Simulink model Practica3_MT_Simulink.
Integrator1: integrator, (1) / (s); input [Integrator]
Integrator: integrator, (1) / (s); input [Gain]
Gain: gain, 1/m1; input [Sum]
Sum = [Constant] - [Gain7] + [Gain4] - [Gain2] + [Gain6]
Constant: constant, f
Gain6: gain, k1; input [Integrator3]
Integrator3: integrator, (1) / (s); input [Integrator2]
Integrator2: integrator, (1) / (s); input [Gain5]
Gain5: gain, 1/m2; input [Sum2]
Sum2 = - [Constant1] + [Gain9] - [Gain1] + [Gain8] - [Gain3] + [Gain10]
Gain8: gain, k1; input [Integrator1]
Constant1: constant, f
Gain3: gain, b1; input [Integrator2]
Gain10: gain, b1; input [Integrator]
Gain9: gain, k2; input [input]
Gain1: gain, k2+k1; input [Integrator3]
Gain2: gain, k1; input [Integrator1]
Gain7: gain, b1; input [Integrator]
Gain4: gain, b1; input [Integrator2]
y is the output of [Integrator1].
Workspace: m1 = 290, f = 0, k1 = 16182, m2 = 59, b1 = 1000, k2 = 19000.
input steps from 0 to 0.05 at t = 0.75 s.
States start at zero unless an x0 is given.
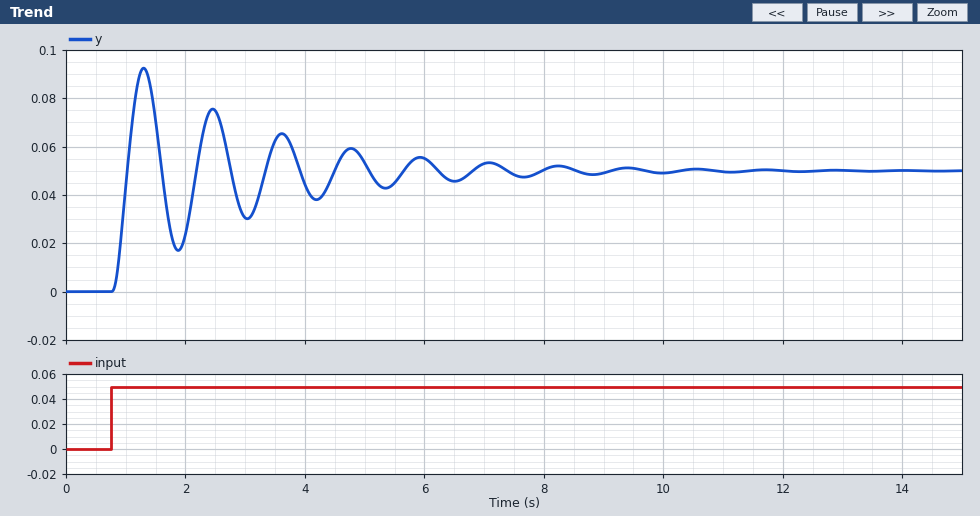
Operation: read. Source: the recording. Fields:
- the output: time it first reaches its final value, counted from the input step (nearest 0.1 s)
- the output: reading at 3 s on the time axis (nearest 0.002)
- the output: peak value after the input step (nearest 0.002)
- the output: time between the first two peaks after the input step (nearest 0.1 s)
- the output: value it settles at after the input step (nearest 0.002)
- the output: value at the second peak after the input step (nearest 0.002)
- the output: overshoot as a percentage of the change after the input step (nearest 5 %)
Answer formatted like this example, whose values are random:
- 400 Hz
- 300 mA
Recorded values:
- 0.3 s
- 0.030
- 0.092
- 1.2 s
- 0.050
- 0.076
- 85 %
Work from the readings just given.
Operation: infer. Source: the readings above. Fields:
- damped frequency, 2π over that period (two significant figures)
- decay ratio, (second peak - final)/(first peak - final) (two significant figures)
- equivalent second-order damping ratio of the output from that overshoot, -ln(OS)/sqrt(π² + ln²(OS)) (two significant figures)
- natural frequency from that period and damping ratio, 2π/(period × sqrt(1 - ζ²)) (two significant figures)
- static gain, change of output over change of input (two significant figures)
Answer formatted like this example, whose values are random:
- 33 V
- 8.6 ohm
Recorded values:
- 5.2 rad/s
- 0.62
- 0.052
- 5.2 rad/s
- 1.0
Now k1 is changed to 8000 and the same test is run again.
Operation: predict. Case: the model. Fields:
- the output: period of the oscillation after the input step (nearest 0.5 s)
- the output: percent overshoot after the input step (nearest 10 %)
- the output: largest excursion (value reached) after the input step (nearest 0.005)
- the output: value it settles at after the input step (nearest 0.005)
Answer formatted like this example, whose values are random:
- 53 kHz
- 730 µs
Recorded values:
- 1.5 s
- 70 %
- 0.085
- 0.050
